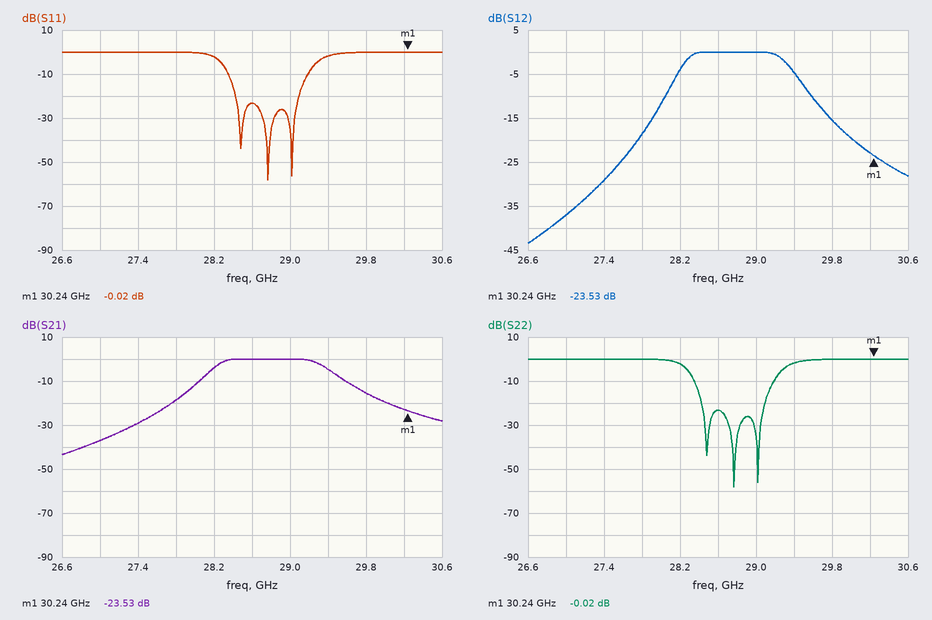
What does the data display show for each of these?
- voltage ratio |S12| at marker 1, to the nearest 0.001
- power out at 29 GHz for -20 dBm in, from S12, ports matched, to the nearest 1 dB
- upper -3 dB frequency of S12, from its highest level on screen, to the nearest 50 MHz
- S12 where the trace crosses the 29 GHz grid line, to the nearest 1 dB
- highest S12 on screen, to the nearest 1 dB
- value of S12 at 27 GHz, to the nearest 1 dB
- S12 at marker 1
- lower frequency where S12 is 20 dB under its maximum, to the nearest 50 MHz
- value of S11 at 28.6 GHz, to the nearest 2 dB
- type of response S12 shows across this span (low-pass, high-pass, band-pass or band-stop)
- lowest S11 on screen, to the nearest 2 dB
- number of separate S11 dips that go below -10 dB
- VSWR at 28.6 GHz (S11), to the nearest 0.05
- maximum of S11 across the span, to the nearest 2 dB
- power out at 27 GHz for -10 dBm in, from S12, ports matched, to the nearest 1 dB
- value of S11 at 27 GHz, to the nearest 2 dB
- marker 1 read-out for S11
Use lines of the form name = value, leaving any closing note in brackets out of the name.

voltage ratio |S12| at marker 1, to the nearest 0.001 = 0.067
power out at 29 GHz for -20 dBm in, from S12, ports matched, to the nearest 1 dB = -20 dBm
upper -3 dB frequency of S12, from its highest level on screen, to the nearest 50 MHz = 29.35 GHz
S12 where the trace crosses the 29 GHz grid line, to the nearest 1 dB = 0 dB
highest S12 on screen, to the nearest 1 dB = 0 dB
value of S12 at 27 GHz, to the nearest 1 dB = -37 dB
S12 at marker 1 = -23.53 dB
lower frequency where S12 is 20 dB under its maximum, to the nearest 50 MHz = 27.75 GHz
value of S11 at 28.6 GHz, to the nearest 2 dB = -24 dB
type of response S12 shows across this span = band-pass
lowest S11 on screen, to the nearest 2 dB = -58 dB
number of separate S11 dips that go below -10 dB = 3
VSWR at 28.6 GHz (S11), to the nearest 0.05 = 1.15
maximum of S11 across the span, to the nearest 2 dB = 0 dB
power out at 27 GHz for -10 dBm in, from S12, ports matched, to the nearest 1 dB = -47 dBm
value of S11 at 27 GHz, to the nearest 2 dB = 0 dB
marker 1 read-out for S11 = -0.02 dB
